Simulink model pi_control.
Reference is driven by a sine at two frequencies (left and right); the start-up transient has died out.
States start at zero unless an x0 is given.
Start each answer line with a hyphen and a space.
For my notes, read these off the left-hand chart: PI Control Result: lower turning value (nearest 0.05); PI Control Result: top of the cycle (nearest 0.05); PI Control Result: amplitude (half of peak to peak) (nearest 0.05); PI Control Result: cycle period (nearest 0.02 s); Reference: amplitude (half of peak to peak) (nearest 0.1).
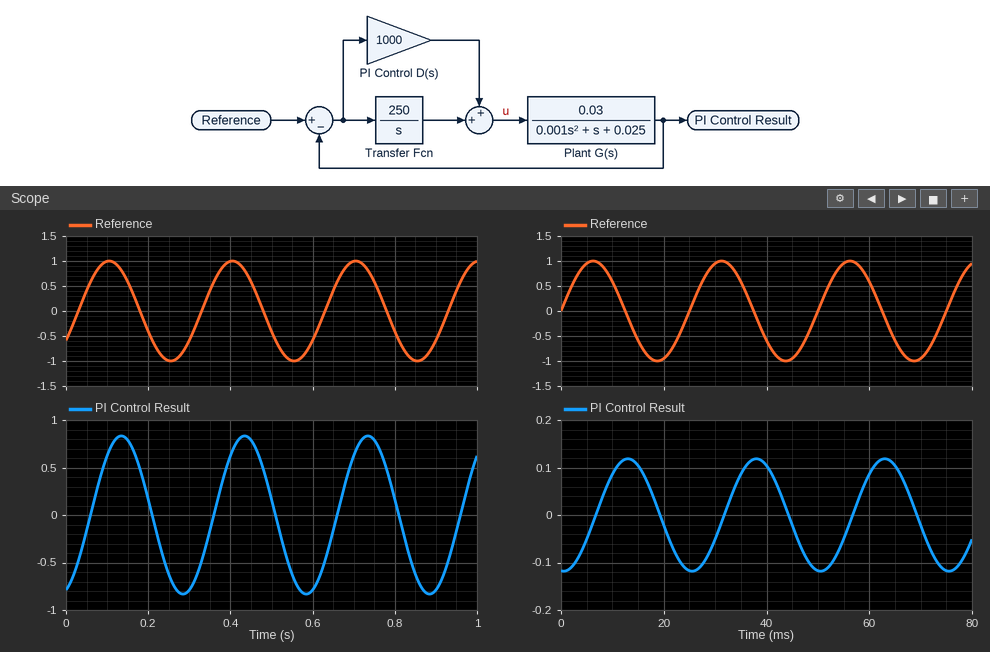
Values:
- -0.85
- 0.85
- 0.85
- 0.30 s
- 1.0
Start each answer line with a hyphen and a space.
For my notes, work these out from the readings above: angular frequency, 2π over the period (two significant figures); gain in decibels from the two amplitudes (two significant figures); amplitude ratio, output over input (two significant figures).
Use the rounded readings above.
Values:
- 21 rad/s
- -1.4 dB
- 0.85
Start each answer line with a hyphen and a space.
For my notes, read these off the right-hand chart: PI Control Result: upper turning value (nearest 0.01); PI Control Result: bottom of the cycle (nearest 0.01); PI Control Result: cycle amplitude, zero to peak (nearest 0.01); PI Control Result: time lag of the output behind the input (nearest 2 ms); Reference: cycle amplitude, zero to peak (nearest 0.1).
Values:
- 0.12
- -0.12
- 0.12
- 6 ms
- 1.0
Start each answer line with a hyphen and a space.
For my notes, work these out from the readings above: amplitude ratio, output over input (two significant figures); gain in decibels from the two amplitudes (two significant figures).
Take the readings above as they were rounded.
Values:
- 0.12
- -18 dB
